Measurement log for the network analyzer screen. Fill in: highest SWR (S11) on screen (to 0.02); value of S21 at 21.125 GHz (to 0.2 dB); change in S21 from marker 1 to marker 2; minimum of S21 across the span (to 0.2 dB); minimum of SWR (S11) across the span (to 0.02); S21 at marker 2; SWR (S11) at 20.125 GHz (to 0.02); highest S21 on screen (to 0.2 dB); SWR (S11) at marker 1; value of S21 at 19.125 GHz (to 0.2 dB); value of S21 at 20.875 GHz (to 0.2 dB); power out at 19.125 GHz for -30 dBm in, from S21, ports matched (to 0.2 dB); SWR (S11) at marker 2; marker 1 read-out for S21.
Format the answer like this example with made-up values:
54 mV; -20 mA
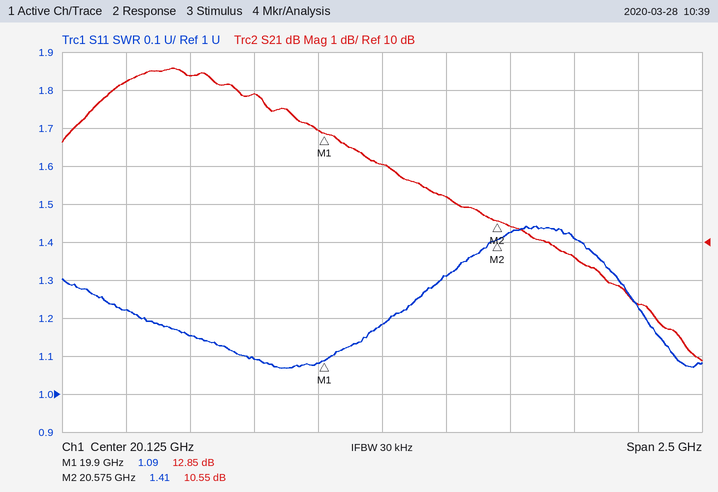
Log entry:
1.44; 8.4 dB; -2.30 dB; 6.8 dB; 1.06; 10.55 dB; 1.18; 14.6 dB; 1.09; 14.2 dB; 9.6 dB; -15.8 dBm; 1.41; 12.85 dB
